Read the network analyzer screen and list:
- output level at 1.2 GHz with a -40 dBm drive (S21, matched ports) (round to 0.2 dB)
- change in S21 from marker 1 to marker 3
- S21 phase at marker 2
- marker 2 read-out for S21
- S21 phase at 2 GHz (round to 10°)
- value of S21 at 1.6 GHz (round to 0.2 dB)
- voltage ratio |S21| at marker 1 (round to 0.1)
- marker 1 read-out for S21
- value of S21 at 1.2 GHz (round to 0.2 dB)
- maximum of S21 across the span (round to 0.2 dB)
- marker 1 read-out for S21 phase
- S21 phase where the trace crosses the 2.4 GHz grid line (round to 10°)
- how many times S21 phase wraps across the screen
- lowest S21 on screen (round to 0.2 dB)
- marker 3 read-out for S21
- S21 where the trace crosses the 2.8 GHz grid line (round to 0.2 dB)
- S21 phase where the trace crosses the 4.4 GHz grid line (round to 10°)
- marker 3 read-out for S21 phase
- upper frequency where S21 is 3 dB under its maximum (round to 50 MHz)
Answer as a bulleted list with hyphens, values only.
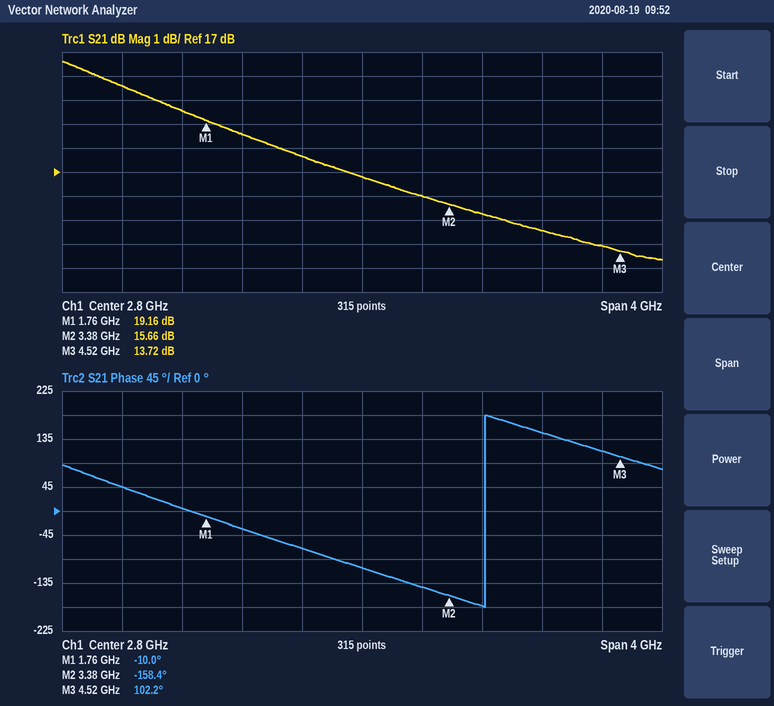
- -19.4 dBm
- -5.44 dB
- -158.4°
- 15.66 dB
- -30°
- 19.6 dB
- 9.1
- 19.16 dB
- 20.6 dB
- 21.6 dB
- -10.0°
- -70°
- 1
- 13.4 dB
- 13.72 dB
- 16.8 dB
- 110°
- 102.2°
- 2.00 GHz
